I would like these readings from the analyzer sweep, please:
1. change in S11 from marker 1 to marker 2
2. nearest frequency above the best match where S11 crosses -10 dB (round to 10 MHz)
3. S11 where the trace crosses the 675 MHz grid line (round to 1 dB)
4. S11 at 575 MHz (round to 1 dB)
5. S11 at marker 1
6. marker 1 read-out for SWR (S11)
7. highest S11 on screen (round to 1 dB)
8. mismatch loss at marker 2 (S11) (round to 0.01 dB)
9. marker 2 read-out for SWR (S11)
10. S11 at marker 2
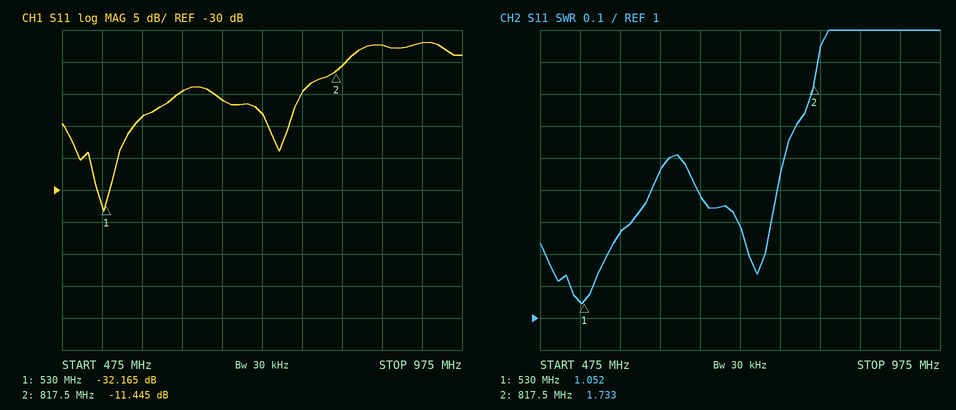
20.720 dB
830 MHz
-16 dB
-19 dB
-32.165 dB
1.052
-7 dB
0.32 dB
1.733
-11.445 dB
